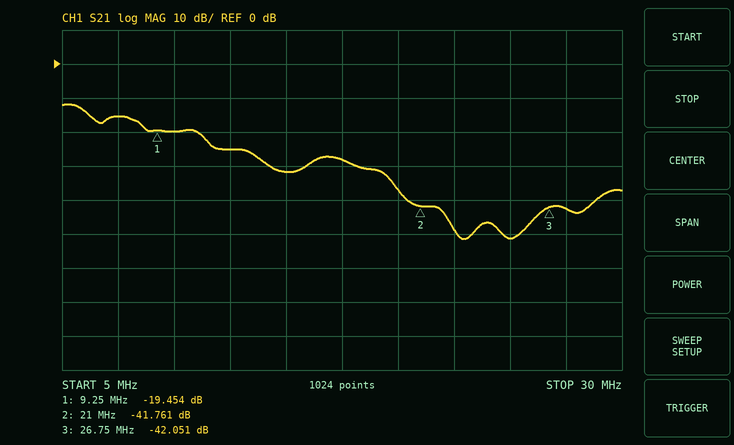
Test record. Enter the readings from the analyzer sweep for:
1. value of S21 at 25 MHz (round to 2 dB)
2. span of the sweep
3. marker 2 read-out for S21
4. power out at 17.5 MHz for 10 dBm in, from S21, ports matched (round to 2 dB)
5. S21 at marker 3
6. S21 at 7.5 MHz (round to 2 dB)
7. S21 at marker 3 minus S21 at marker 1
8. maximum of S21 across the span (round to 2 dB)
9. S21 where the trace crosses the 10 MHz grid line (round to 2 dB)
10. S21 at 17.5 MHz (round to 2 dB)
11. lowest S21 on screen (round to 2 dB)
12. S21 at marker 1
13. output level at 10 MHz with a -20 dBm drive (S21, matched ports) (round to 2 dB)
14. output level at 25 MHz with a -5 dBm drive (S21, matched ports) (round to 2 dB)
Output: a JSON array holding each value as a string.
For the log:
["-52 dB", "25 MHz", "-41.761 dB", "-18 dBm", "-42.051 dB", "-16 dB", "-22.597 dB", "-12 dB", "-20 dB", "-28 dB", "-52 dB", "-19.454 dB", "-40 dBm", "-56 dBm"]
